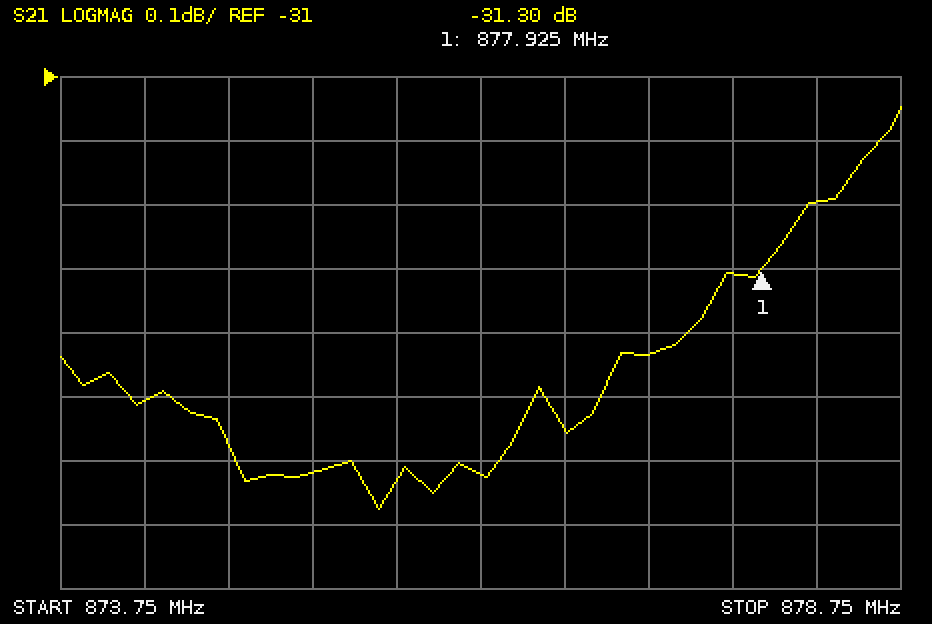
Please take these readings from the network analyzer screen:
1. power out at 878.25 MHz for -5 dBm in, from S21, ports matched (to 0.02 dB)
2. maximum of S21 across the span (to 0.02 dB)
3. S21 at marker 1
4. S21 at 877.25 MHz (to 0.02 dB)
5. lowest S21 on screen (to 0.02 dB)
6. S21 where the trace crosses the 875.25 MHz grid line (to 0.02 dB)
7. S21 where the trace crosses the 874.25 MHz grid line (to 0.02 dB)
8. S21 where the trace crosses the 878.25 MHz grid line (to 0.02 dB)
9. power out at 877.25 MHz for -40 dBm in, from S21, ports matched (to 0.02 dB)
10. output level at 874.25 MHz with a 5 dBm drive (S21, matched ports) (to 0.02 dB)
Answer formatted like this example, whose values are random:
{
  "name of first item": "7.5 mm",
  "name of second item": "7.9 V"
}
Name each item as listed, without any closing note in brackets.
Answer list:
{
  "power out at 878.25 MHz for -5 dBm in, from S21, ports matched": "-36.20 dBm",
  "maximum of S21 across the span": "-31.04 dB",
  "S21 at marker 1": "-31.30 dB",
  "S21 at 877.25 MHz": "-31.44 dB",
  "lowest S21 on screen": "-31.68 dB",
  "S21 where the trace crosses the 875.25 MHz grid line": "-31.62 dB",
  "S21 where the trace crosses the 874.25 MHz grid line": "-31.50 dB",
  "S21 where the trace crosses the 878.25 MHz grid line": "-31.20 dB",
  "power out at 877.25 MHz for -40 dBm in, from S21, ports matched": "-71.44 dBm",
  "output level at 874.25 MHz with a 5 dBm drive (S21, matched ports)": "-26.50 dBm"
}
